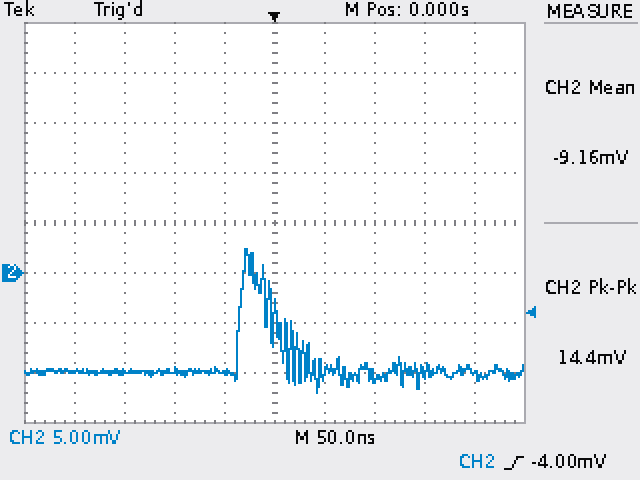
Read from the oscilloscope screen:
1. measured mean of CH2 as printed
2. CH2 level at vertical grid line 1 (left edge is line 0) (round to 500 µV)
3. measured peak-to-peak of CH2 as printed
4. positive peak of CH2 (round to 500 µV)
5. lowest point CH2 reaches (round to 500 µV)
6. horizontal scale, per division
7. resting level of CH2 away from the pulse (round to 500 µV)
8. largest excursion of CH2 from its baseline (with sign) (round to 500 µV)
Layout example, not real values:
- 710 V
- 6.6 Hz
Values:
- -9.16 mV
- -10.0 mV
- 14.4 mV
- 2.5 mV
- -12.0 mV
- 50 ns
- -10.0 mV
- +12.5 mV
